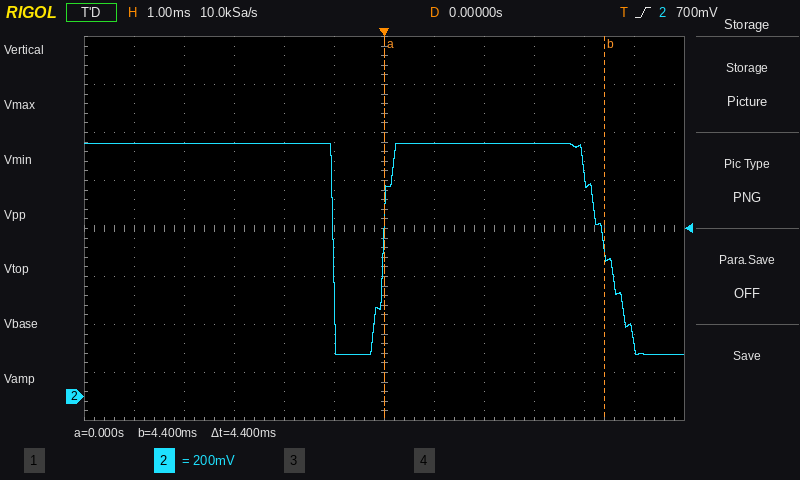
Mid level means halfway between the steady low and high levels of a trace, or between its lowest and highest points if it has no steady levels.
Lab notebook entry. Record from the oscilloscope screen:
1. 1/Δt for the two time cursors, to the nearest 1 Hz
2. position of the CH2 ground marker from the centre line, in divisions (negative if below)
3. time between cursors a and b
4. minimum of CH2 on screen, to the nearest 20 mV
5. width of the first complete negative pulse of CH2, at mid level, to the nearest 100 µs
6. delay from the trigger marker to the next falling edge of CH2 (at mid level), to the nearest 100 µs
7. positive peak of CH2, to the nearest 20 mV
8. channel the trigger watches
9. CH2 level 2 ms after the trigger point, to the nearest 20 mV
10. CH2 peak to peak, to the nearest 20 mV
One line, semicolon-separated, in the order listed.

227 Hz; -3.5 div; 4.4 ms; 180 mV; 1.0 ms; 4.4 ms; 1.06 V; CH2; 1.06 V; 880 mV
